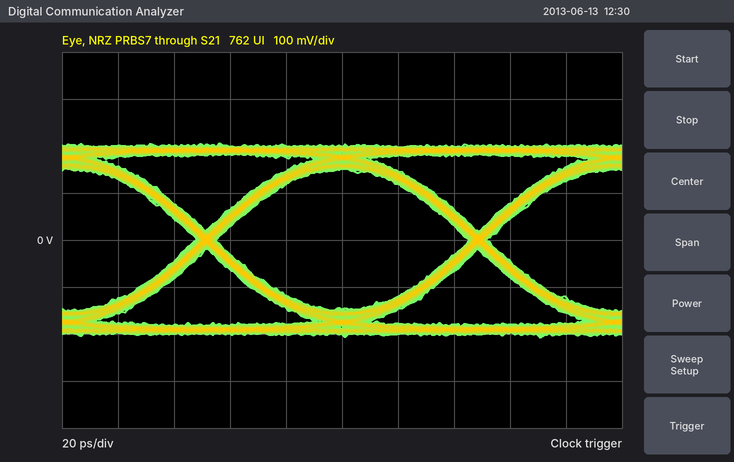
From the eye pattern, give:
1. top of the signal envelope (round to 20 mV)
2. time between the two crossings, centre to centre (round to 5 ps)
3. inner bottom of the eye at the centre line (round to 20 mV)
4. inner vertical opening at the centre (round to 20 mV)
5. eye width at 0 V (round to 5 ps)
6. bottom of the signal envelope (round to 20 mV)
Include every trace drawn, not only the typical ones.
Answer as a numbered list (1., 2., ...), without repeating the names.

1. 200 mV
2. 95 ps
3. -140 mV
4. 300 mV
5. 90 ps
6. -200 mV
